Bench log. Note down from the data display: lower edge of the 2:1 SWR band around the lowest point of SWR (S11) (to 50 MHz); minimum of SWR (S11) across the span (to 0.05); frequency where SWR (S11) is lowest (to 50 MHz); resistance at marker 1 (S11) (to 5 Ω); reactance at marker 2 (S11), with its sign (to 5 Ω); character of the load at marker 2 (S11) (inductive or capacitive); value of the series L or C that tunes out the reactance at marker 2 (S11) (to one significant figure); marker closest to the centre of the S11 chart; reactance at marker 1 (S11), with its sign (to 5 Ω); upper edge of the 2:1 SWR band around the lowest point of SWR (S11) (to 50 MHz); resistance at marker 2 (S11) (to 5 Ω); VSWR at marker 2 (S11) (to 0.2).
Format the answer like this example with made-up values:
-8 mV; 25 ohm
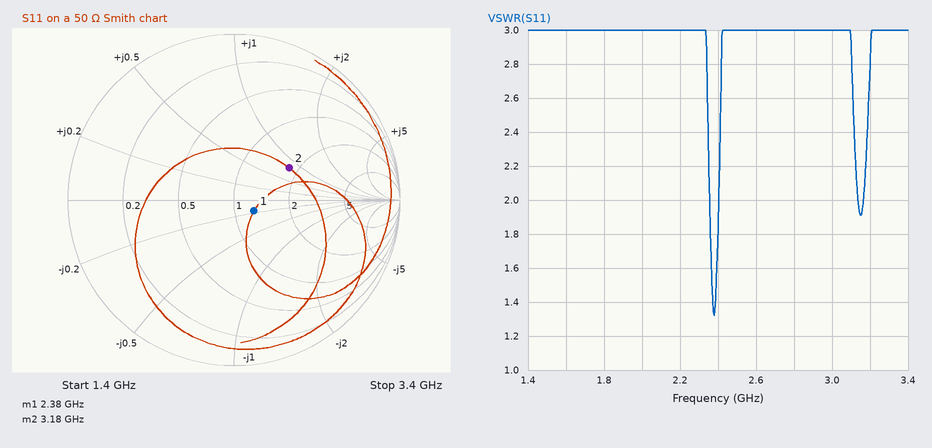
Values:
2.35 GHz; 1.30; 2.40 GHz; 65 Ω; +40 Ω; inductive; 1 pF; marker 1; -10 Ω; 2.40 GHz; 90 Ω; 2.2
